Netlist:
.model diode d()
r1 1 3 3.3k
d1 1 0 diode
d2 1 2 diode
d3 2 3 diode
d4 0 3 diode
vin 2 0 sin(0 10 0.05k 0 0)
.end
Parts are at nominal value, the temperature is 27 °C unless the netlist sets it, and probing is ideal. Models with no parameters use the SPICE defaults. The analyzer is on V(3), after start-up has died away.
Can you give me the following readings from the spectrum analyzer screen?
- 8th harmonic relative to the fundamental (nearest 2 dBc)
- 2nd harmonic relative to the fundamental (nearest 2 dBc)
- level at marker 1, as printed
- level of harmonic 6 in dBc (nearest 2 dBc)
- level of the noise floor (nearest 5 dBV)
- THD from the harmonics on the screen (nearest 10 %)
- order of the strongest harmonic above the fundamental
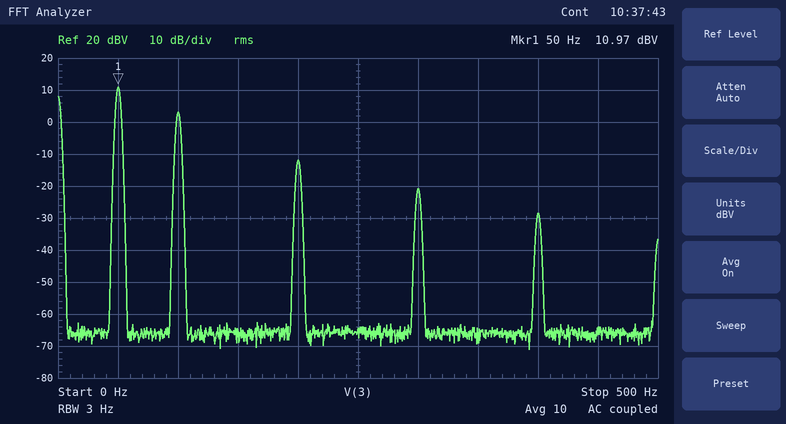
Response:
-40 dBc
-8 dBc
10.97 dBV
-32 dBc
-65 dBV
40 %
2
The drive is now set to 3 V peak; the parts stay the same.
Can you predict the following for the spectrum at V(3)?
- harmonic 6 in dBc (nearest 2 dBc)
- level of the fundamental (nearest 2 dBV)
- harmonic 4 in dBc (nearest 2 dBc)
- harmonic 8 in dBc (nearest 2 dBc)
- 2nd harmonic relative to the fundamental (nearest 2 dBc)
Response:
-34 dBc
0 dBV
-50 dBc
-36 dBc
-10 dBc
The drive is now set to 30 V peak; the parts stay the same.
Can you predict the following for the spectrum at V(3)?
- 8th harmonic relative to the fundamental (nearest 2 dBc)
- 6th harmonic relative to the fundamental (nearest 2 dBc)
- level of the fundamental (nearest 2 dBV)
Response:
-34 dBc
-30 dBc
20 dBV
